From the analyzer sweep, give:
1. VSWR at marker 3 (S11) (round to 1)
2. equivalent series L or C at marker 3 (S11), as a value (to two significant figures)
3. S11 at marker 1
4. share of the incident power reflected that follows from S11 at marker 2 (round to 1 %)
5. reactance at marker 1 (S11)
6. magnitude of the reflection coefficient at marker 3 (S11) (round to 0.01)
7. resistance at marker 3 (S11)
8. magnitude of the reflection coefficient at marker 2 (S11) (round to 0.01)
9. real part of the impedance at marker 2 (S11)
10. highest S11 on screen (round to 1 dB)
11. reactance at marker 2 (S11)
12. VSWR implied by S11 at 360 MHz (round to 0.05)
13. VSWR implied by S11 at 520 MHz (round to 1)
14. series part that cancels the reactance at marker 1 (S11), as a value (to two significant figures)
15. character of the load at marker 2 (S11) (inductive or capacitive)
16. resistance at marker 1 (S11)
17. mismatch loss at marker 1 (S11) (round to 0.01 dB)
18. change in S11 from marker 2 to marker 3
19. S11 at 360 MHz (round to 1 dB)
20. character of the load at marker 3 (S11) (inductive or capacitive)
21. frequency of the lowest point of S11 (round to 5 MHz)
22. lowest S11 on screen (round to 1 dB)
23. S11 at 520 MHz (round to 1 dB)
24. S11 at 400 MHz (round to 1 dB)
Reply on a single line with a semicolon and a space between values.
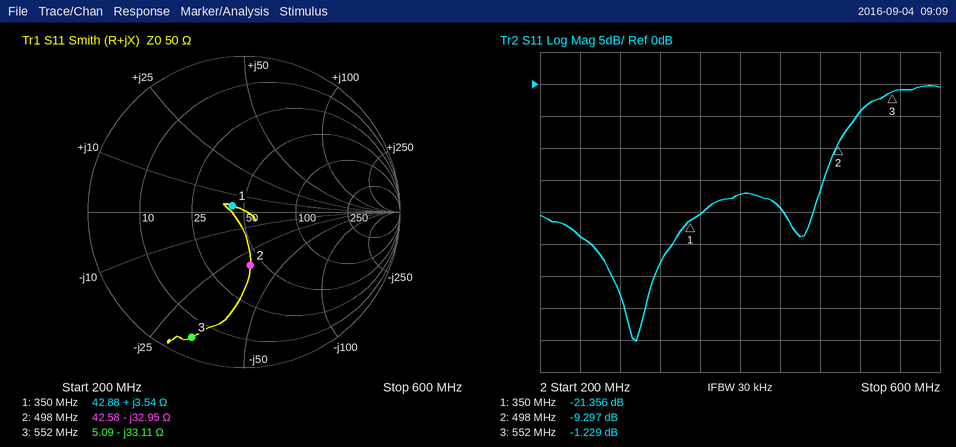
14; 8.7 pF; -21.356 dB; 12 %; +3.54 Ω; 0.87; 5.09 Ω; 0.34; 42.58 Ω; 0 dB; -32.95 Ω; 1.20; 4; 130 pF; capacitive; 42.88 Ω; 0.03 dB; 8.068 dB; -20 dB; capacitive; 295 MHz; -40 dB; -4 dB; -17 dB
